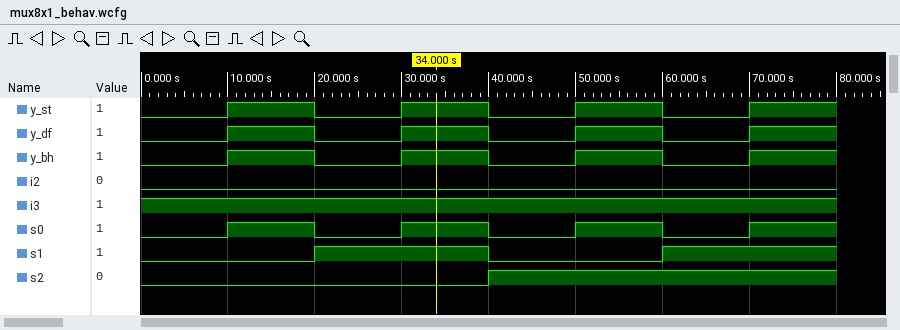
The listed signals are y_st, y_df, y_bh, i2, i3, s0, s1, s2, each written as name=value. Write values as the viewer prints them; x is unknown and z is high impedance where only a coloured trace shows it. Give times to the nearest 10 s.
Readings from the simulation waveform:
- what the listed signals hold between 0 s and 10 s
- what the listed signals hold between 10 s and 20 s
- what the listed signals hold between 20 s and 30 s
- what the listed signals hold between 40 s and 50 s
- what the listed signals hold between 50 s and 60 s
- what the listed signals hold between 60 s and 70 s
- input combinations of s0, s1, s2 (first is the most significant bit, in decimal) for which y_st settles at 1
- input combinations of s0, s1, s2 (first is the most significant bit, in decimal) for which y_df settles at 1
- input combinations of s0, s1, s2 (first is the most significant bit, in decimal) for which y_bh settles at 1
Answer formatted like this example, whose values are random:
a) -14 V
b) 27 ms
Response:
a) y_st=0, y_df=0, y_bh=0, i2=0, i3=1, s0=0, s1=0, s2=0
b) y_st=1, y_df=1, y_bh=1, i2=0, i3=1, s0=1, s1=0, s2=0
c) y_st=0, y_df=0, y_bh=0, i2=0, i3=1, s0=0, s1=1, s2=0
d) y_st=0, y_df=0, y_bh=0, i2=0, i3=1, s0=0, s1=0, s2=1
e) y_st=1, y_df=1, y_bh=1, i2=0, i3=1, s0=1, s1=0, s2=1
f) y_st=0, y_df=0, y_bh=0, i2=0, i3=1, s0=0, s1=1, s2=1
g) 4, 5, 6, 7
h) 4, 5, 6, 7
i) 4, 5, 6, 7
